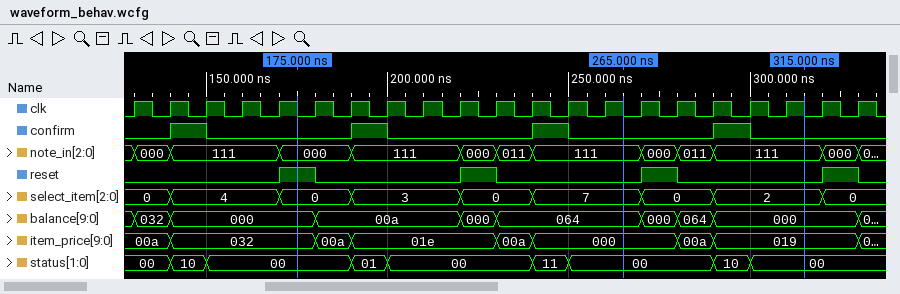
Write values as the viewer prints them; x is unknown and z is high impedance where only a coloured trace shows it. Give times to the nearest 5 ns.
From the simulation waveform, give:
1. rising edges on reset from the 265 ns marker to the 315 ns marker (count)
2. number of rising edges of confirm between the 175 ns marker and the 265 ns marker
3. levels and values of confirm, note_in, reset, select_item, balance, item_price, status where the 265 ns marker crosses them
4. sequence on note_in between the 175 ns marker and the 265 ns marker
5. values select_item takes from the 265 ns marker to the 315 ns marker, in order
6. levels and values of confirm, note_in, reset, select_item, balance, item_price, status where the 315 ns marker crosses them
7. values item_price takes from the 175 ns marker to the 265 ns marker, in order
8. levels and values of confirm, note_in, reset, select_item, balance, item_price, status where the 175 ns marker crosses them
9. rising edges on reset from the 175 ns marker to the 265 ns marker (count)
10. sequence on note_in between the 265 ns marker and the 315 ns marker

1
2
confirm=0, note_in=111, reset=0, select_item=7, balance=064, item_price=000, status=00
000, 111, 000, 011, 111
7, 0, 2
confirm=0, note_in=111, reset=0, select_item=2, balance=000, item_price=019, status=00
032, 00a, 01e, 00a, 000
confirm=0, note_in=000, reset=1, select_item=0, balance=000, item_price=032, status=00
1
111, 000, 011, 111
